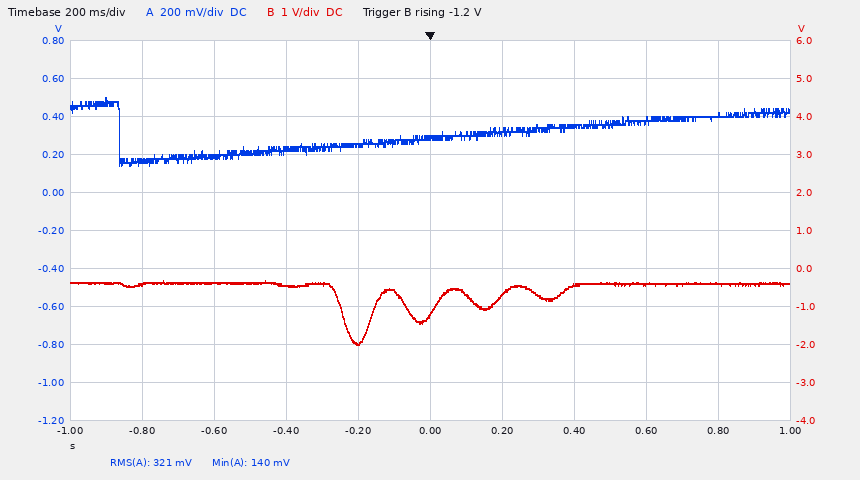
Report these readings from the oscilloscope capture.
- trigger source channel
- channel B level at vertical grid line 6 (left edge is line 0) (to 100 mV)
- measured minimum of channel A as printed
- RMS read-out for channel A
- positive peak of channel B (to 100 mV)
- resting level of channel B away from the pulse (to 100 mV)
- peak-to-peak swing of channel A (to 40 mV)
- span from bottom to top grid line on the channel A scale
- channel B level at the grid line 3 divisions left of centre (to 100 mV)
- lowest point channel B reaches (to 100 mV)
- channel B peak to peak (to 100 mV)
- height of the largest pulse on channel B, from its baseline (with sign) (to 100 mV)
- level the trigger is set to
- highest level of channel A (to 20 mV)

channel B
-700 mV
140 mV
321 mV
-300 mV
-400 mV
360 mV
2 V
-400 mV
-2.0 V
1.7 V
-1.6 V
-1.2 V
500 mV
